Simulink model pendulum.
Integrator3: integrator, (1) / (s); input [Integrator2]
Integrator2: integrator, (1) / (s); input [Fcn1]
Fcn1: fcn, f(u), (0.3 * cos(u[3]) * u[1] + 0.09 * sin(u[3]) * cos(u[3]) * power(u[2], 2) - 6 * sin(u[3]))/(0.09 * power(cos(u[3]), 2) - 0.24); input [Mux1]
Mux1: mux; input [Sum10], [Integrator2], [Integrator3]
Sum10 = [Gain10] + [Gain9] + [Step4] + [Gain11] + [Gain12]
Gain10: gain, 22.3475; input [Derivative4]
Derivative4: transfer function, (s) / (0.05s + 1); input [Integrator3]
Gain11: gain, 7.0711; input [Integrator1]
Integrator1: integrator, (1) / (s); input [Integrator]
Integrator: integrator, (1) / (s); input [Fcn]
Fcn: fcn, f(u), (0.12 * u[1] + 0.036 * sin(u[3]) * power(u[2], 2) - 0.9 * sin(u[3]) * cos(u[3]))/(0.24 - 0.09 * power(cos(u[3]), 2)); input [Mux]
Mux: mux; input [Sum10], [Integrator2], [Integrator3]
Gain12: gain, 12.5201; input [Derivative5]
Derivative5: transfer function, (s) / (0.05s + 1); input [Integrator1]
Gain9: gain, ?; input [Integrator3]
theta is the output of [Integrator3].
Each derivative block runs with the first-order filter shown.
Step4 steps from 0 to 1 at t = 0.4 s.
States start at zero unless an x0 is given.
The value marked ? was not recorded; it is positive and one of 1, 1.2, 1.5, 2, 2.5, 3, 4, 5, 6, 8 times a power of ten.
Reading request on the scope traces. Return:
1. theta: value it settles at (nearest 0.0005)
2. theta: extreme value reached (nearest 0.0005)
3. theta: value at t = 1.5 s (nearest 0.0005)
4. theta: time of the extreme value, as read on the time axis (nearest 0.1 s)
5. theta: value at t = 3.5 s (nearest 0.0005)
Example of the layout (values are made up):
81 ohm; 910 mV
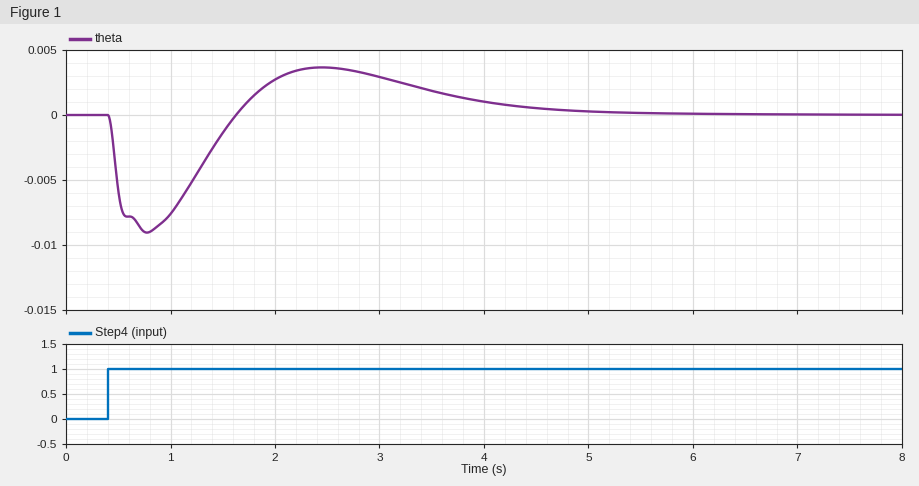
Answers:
0.0000; -0.0090; -0.0015; 0.8 s; 0.0020
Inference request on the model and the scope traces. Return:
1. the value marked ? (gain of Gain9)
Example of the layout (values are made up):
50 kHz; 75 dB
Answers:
100
